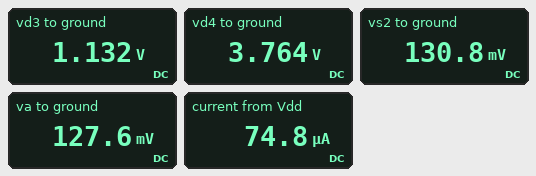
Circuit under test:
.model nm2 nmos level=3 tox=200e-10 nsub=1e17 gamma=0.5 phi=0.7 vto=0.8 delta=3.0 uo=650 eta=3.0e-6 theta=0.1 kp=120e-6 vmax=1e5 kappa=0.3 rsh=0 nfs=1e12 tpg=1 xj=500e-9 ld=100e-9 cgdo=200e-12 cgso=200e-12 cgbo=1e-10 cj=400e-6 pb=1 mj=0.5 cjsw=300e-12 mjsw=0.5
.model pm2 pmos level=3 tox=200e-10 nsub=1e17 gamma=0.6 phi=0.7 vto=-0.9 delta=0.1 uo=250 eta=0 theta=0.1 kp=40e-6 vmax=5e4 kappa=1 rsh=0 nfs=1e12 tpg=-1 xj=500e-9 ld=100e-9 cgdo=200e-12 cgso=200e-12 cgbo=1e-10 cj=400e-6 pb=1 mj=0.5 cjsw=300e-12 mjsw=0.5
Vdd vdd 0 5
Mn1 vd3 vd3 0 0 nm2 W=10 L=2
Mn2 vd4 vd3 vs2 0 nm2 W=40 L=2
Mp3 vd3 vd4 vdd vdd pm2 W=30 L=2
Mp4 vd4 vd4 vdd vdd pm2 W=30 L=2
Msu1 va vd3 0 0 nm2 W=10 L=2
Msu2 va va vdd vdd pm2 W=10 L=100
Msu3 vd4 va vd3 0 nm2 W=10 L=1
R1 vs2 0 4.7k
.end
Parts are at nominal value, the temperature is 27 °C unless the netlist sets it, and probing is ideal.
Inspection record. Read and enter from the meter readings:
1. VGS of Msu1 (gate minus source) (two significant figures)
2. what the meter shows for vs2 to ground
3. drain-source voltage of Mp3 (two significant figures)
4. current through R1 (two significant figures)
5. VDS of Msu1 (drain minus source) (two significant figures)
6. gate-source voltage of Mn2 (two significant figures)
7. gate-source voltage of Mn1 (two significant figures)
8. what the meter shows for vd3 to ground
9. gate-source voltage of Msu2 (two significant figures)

1.1 V
130.8 mV
-3.9 V
28 µA
130 mV
1.0 V
1.1 V
1.132 V
-4.9 V
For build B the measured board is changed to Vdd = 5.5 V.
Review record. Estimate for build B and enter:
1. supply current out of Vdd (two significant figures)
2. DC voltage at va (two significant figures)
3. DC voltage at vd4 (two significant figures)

79 µA
170 mV
4.3 V
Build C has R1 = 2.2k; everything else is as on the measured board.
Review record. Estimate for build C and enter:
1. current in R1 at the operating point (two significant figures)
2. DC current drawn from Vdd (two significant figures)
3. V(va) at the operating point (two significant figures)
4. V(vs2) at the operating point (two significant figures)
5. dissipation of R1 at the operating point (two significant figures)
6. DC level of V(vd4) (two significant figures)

140 µA
300 µA
49 mV
310 mV
43 µW
3.3 V
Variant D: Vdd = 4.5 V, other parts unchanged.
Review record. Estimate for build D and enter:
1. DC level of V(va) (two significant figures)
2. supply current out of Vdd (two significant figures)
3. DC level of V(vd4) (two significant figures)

96 mV
71 µA
3.3 V
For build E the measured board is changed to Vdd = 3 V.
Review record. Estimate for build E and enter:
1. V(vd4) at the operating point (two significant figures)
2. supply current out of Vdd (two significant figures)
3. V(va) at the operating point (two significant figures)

1.8 V
62 µA
33 mV
